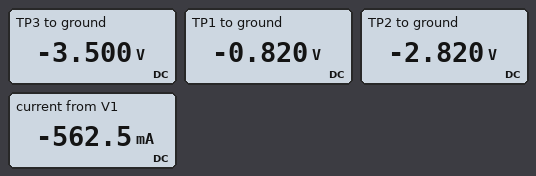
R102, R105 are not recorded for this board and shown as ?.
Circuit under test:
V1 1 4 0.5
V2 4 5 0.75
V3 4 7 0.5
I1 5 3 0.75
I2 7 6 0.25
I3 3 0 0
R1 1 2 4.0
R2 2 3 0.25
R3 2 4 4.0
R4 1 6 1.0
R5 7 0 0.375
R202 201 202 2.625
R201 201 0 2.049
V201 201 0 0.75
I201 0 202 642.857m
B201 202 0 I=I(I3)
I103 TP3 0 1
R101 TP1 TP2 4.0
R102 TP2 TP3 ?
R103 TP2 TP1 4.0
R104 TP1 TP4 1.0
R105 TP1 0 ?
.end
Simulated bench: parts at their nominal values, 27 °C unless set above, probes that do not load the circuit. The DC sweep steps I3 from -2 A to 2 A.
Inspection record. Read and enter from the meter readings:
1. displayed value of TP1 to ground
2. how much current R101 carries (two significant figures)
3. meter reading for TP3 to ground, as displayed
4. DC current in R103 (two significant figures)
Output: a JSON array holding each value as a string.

["-0.820 V", "500 mA", "-3.500 V", "500 mA"]
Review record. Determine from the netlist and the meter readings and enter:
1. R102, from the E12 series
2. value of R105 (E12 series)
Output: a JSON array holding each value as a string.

["0.68 Ω", "0.82 Ω"]
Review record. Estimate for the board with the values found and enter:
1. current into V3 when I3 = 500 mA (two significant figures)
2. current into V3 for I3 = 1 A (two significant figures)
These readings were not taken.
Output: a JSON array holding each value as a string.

["-250 mA", "-750 mA"]
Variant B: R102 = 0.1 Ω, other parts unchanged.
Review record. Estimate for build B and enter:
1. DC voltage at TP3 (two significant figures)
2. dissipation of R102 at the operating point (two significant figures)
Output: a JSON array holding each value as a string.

["-2.9 V", "100 mW"]
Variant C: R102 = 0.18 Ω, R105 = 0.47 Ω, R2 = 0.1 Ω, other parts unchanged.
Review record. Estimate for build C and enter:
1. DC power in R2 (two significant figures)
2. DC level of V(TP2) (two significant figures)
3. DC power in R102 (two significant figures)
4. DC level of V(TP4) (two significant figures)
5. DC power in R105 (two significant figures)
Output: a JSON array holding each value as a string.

["56 mW", "-2.5 V", "180 mW", "-470 mV", "470 mW"]
